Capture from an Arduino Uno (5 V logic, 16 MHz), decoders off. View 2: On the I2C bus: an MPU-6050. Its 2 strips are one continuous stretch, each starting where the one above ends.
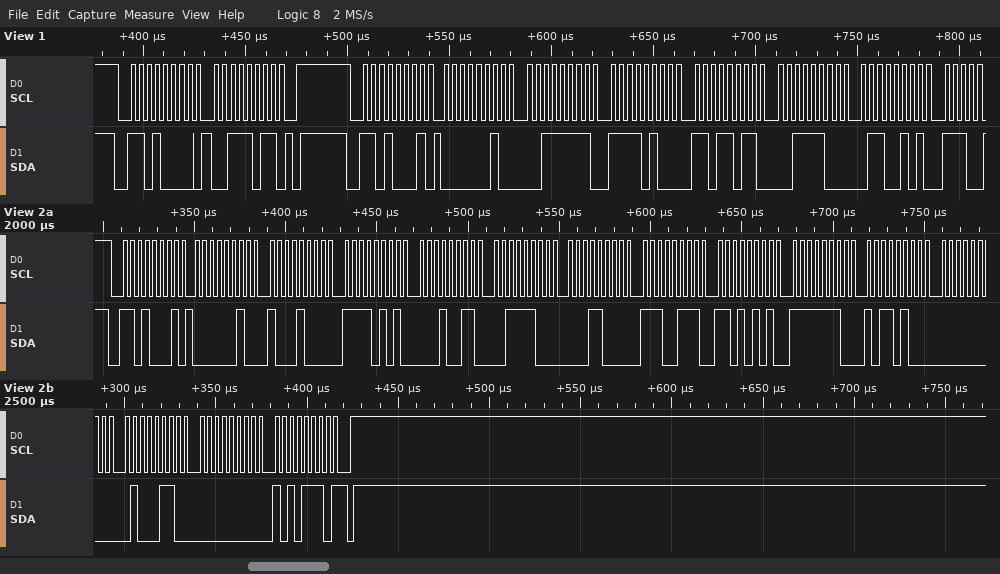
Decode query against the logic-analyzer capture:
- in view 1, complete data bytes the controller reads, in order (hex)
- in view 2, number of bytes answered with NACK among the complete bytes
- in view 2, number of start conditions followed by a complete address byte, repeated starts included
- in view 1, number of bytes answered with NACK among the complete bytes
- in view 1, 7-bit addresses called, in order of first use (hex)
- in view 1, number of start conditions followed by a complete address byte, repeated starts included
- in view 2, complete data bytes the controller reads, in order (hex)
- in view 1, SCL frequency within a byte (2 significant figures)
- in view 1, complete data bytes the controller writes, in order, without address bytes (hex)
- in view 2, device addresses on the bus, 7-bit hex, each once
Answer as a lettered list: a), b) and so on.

a) 02 3F F4 DB 3C 65
b) 1
c) 1
d) 0
e) 0x68
f) 2
g) 02 88 F5 13 3C 18 E7 D5 FE B4 00 46 00 AE
h) 250 kHz
i) 3B
j) 0x68
